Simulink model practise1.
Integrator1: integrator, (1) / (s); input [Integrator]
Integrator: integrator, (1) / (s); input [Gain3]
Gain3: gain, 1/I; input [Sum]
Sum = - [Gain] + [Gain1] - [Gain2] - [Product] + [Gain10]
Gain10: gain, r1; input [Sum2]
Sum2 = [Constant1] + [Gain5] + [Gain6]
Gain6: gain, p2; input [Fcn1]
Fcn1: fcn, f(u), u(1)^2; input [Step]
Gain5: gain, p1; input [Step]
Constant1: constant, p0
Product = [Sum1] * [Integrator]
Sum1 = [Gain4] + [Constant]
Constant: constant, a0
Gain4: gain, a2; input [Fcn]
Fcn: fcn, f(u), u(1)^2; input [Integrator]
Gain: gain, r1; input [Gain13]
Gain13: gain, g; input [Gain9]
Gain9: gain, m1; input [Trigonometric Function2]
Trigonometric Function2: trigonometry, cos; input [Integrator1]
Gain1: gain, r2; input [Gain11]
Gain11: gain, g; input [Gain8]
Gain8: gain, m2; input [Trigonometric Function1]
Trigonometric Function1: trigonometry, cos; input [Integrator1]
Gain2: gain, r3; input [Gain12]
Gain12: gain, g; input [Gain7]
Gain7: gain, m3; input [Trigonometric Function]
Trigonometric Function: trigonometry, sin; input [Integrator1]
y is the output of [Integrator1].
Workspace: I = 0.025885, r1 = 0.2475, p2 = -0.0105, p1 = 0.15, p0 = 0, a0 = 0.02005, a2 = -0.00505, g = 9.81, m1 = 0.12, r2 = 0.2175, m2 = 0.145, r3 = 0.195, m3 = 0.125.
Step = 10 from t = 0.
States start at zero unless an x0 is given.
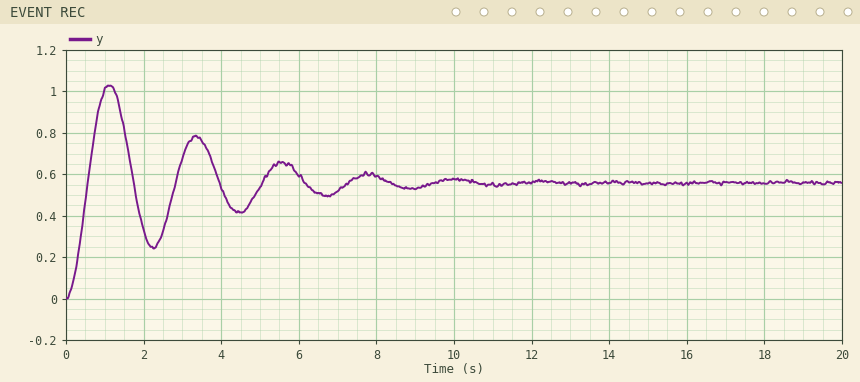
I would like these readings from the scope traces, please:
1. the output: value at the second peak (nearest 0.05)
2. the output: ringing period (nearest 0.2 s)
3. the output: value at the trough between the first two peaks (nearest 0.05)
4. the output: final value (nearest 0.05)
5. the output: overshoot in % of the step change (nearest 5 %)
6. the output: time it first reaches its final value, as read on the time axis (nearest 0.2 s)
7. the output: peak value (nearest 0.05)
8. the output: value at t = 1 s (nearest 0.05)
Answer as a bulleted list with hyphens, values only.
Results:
- 0.80
- 2.2 s
- 0.25
- 0.55
- 85 %
- 0.6 s
- 1.05
- 1.00
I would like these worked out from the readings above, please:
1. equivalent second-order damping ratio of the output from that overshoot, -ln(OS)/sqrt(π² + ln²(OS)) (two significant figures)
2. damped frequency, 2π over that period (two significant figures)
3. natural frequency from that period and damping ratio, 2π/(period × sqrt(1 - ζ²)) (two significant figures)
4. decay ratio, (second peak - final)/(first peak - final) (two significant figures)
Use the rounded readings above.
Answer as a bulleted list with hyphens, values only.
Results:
- 0.052
- 2.9 rad/s
- 2.9 rad/s
- 0.50
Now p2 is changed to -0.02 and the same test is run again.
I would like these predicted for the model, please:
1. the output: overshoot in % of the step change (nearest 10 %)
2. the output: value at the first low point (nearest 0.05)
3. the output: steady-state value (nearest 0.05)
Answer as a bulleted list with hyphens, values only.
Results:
- 80 %
- -0.85
- -0.45
